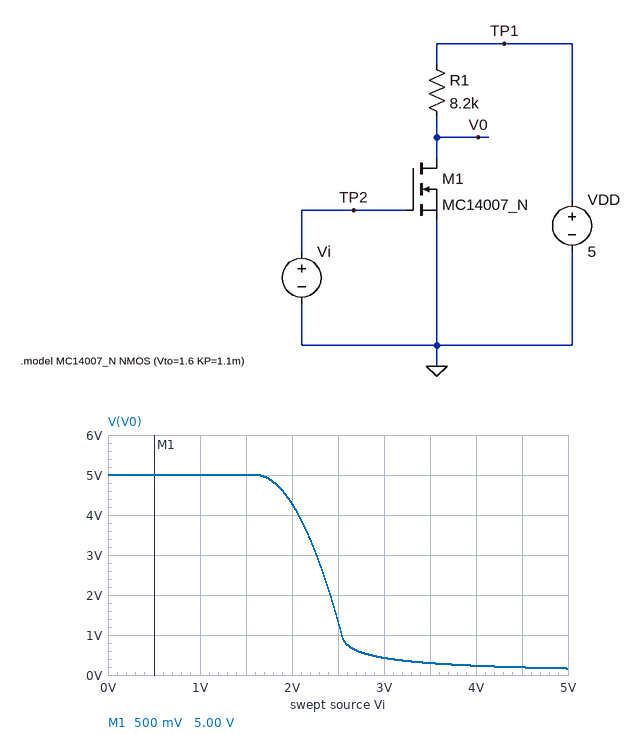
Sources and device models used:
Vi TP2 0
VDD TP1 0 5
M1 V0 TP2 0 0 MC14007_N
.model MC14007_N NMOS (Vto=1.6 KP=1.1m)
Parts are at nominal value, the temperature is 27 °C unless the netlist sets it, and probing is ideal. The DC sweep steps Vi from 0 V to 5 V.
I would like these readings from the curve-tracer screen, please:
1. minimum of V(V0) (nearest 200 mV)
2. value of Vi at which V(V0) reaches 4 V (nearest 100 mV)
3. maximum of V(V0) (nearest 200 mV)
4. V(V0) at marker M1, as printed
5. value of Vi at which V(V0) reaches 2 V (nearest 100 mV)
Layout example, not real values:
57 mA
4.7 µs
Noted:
200 mV
2.1 V
5.0 V
5.00 V
2.4 V
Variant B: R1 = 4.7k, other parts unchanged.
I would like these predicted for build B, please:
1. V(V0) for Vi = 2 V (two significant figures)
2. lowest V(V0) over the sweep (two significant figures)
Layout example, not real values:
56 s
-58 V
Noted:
4.6 V
280 mV
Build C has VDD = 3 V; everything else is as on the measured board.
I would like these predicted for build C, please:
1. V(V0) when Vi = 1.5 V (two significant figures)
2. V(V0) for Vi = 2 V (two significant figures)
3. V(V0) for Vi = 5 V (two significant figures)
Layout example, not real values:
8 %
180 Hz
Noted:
3.0 V
2.3 V
96 mV
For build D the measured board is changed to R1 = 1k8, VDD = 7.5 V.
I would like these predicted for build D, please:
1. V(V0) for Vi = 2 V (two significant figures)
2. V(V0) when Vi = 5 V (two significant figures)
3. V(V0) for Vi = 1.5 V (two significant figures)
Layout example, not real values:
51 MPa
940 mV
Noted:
7.3 V
1.1 V
7.5 V
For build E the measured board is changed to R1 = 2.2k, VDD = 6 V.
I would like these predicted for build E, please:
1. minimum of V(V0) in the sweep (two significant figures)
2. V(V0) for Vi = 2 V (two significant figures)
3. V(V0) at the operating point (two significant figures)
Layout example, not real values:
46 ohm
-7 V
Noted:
720 mV
5.8 V
6.0 V
